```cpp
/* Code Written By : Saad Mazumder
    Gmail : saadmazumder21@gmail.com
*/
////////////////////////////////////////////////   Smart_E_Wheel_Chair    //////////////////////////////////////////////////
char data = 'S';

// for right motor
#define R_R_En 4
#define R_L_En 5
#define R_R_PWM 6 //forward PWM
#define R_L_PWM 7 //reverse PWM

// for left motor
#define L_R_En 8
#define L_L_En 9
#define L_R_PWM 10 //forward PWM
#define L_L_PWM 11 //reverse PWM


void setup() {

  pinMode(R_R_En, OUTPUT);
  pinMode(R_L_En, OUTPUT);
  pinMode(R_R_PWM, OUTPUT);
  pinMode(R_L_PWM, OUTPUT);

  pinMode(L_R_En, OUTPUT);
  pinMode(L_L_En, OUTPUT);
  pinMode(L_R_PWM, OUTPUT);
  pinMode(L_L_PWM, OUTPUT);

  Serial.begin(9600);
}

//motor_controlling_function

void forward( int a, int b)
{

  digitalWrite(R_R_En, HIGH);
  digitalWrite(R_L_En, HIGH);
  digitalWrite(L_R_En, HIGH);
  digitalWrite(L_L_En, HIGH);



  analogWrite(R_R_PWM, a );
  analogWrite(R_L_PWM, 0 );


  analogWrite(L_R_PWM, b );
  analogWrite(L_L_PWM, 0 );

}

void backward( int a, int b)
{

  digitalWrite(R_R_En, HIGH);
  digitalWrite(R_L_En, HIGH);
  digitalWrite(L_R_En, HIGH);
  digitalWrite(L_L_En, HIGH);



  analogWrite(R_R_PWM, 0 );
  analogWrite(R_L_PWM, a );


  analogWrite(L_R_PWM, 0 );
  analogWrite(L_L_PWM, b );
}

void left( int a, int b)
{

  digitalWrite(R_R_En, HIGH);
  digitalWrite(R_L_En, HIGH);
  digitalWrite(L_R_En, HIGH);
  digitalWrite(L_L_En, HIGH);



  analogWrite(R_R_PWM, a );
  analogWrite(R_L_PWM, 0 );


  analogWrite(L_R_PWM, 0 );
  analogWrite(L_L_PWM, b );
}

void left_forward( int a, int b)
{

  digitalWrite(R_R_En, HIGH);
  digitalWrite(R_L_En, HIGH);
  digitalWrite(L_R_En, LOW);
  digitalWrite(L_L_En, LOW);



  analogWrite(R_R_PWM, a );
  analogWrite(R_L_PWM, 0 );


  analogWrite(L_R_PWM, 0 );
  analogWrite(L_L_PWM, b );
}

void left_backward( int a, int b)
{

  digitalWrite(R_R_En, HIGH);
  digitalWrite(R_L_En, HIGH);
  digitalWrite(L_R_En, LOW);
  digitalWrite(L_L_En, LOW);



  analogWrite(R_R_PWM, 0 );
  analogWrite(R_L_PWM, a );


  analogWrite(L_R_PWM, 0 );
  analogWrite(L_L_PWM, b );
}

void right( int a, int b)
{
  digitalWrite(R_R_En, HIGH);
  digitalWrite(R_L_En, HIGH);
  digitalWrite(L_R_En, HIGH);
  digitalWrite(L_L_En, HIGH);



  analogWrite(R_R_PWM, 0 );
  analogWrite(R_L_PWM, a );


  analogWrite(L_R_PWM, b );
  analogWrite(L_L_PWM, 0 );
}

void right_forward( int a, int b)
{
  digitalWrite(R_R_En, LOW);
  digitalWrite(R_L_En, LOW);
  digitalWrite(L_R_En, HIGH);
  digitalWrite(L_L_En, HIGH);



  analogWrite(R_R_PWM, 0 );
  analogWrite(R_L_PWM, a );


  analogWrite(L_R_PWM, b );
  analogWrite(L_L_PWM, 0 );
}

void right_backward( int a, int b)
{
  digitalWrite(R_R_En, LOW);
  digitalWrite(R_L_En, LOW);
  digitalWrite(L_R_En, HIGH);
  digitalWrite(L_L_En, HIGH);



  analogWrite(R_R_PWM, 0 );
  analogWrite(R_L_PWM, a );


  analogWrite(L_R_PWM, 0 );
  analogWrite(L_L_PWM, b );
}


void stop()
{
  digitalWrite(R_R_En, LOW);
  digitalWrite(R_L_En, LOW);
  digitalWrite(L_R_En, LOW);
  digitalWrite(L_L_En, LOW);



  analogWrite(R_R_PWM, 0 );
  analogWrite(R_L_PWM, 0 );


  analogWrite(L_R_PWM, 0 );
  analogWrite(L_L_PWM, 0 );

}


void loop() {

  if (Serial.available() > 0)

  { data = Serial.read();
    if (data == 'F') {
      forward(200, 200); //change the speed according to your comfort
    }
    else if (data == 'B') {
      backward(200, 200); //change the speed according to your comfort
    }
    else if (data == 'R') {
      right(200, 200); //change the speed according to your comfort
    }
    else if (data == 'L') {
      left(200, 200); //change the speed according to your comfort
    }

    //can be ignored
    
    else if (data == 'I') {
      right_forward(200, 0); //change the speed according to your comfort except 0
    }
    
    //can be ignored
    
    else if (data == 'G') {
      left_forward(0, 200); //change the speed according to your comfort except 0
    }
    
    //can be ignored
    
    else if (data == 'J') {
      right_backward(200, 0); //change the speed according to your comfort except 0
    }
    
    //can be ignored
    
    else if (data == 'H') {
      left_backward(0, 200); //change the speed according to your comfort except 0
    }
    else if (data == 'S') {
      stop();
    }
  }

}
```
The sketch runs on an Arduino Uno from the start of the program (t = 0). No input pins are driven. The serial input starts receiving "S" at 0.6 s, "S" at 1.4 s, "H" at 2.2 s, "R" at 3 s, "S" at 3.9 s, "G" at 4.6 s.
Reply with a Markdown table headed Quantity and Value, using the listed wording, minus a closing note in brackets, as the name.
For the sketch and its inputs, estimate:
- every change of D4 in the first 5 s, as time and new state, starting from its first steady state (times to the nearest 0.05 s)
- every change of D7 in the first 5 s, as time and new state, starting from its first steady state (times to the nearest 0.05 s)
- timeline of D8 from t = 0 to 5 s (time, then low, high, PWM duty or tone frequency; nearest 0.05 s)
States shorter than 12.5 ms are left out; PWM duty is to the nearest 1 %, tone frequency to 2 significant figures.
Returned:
| Quantity | Value |
|---|---|
| every change of D4 in the first 5 s, as time and new state, starting from its first steady state | 0 s low; 2.2 s high; 3.9 s low; 4.6 s high |
| every change of D7 in the first 5 s, as time and new state, starting from its first steady state | 0 s low; 3 s high; 3.9 s low |
| timeline of D8 from t = 0 to 5 s | 0 s low; 3 s high; 3.9 s low |
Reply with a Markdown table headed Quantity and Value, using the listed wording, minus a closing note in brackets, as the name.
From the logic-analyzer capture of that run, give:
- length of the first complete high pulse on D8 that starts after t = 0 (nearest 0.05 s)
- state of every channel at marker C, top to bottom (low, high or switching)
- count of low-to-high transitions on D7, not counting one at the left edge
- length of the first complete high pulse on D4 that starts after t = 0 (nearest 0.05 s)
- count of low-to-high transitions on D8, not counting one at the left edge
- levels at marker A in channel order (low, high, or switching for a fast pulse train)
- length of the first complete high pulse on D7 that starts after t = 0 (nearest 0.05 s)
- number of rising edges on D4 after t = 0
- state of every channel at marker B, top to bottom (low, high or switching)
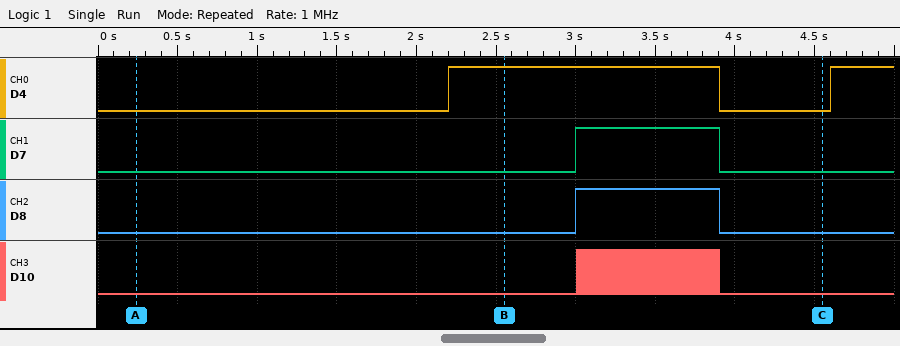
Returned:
| Quantity | Value |
|---|---|
| length of the first complete high pulse on D8 that starts after t = 0 | 0.90 s |
| state of every channel at marker C, top to bottom | D4 low, D7 low, D8 low, D10 low |
| count of low-to-high transitions on D7, not counting one at the left edge | 1 |
| length of the first complete high pulse on D4 that starts after t = 0 | 1.70 s |
| count of low-to-high transitions on D8, not counting one at the left edge | 1 |
| levels at marker A in channel order | D4 low, D7 low, D8 low, D10 low |
| length of the first complete high pulse on D7 that starts after t = 0 | 0.90 s |
| number of rising edges on D4 after t = 0 | 2 |
| state of every channel at marker B, top to bottom | D4 high, D7 low, D8 low, D10 low |
